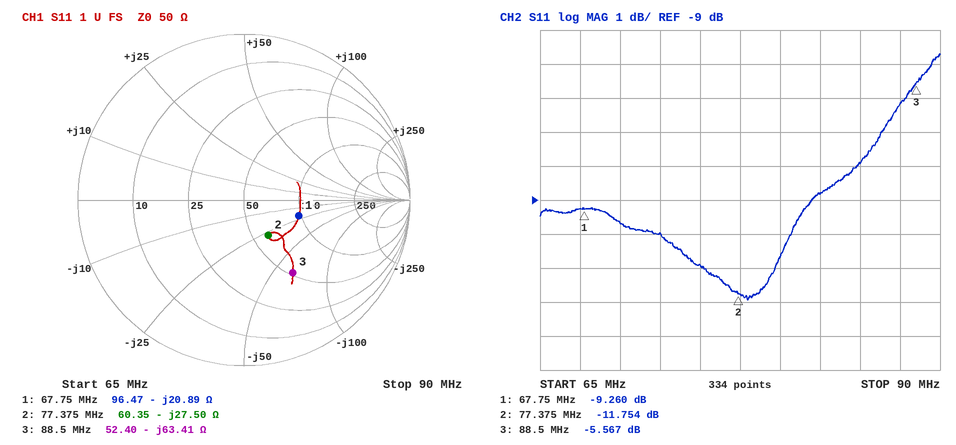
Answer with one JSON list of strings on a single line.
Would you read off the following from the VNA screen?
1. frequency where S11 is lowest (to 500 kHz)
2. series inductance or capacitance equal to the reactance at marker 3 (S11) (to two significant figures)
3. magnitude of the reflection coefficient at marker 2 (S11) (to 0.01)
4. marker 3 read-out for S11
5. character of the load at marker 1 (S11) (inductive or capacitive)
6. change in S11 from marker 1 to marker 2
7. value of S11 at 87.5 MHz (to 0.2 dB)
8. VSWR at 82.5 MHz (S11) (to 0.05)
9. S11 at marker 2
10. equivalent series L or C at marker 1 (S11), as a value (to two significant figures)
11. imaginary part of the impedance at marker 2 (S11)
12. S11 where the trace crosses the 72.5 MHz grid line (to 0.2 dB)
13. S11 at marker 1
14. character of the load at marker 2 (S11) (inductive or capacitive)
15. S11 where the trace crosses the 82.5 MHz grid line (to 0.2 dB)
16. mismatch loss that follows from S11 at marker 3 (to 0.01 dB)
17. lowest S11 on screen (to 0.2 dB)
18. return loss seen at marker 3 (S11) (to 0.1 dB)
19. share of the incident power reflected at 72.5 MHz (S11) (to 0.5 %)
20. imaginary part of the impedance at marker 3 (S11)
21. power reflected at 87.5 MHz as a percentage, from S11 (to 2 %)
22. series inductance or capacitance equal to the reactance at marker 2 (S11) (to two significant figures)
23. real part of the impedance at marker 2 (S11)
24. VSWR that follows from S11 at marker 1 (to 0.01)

["78.0 MHz", "28 pF", "0.26", "-5.567 dB", "capacitive", "-2.494 dB", "-6.2 dB", "2.15", "-11.754 dB", "110 pF", "-27.50 Ω", "-10.0 dB", "-9.260 dB", "capacitive", "-8.8 dB", "1.41 dB", "-12.0 dB", "5.6 dB", "10.0 %", "-63.41 Ω", "24 %", "75 pF", "60.35 Ω", "2.05"]
